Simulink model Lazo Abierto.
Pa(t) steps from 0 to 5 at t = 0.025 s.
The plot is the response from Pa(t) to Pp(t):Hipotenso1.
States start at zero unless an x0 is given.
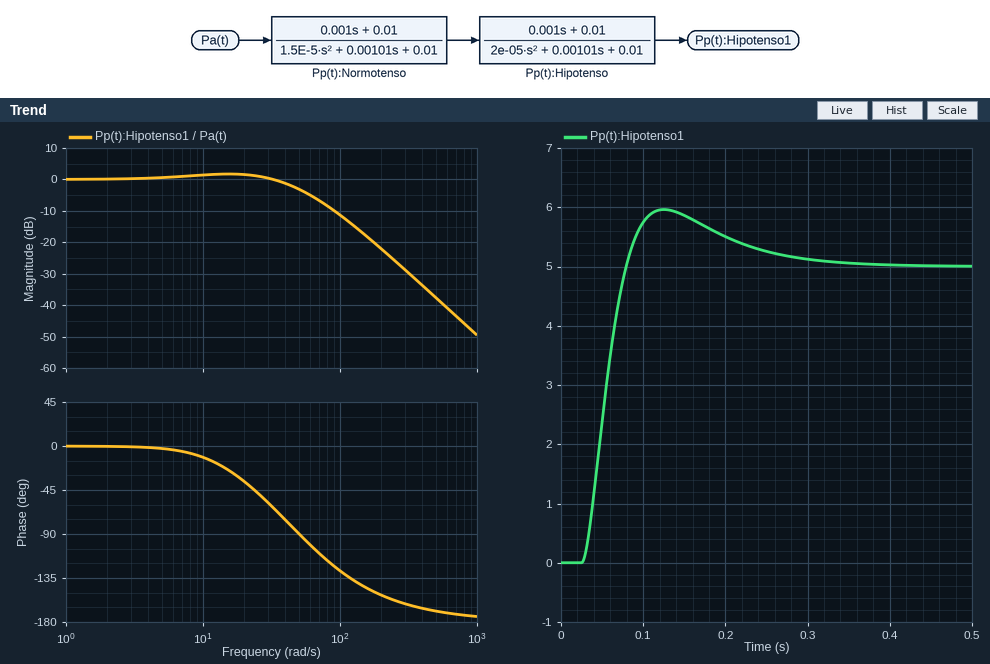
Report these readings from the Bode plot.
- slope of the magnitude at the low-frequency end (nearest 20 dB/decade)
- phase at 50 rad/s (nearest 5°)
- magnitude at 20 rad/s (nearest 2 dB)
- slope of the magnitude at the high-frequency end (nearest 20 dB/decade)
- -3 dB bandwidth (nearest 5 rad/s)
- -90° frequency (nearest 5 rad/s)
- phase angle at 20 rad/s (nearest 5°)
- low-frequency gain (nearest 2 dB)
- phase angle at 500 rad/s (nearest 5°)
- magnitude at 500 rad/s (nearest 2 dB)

0 dB/decade
-90°
2 dB
-40 dB/decade
50 rad/s
50 rad/s
-35°
0 dB
-170°
-38 dB
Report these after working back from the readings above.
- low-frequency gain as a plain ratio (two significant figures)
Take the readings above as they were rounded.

1.0
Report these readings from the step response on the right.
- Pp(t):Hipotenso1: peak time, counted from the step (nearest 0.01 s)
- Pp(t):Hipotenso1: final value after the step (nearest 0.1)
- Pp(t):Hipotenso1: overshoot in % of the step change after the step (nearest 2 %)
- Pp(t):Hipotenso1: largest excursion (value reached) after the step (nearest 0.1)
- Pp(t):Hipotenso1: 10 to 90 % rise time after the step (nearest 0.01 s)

0.10 s
5.0
20 %
6.0
0.04 s
